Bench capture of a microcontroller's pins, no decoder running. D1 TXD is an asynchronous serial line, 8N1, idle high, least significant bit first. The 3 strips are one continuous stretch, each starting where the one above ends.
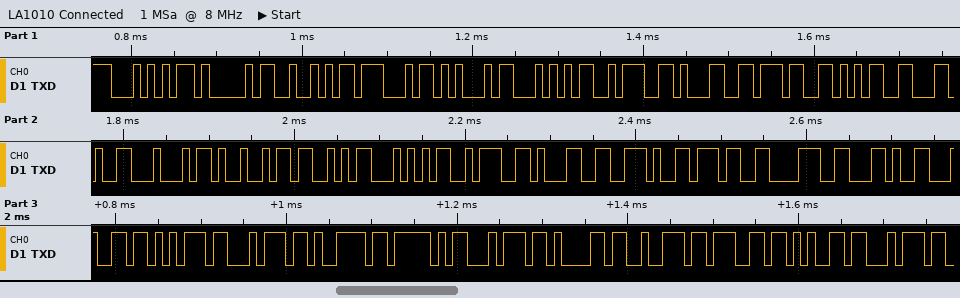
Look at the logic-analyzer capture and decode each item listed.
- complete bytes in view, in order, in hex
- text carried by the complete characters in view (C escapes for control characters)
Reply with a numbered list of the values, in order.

1. 54 41 52 47 45 54 3A 31 37 35 2C 44 49 53 54 3A 31 2E 37 38 2C 64 75 74 79 5F 74 61 72 67 65 74
2. "TARGET:175,DIST:1.78,duty_target"
